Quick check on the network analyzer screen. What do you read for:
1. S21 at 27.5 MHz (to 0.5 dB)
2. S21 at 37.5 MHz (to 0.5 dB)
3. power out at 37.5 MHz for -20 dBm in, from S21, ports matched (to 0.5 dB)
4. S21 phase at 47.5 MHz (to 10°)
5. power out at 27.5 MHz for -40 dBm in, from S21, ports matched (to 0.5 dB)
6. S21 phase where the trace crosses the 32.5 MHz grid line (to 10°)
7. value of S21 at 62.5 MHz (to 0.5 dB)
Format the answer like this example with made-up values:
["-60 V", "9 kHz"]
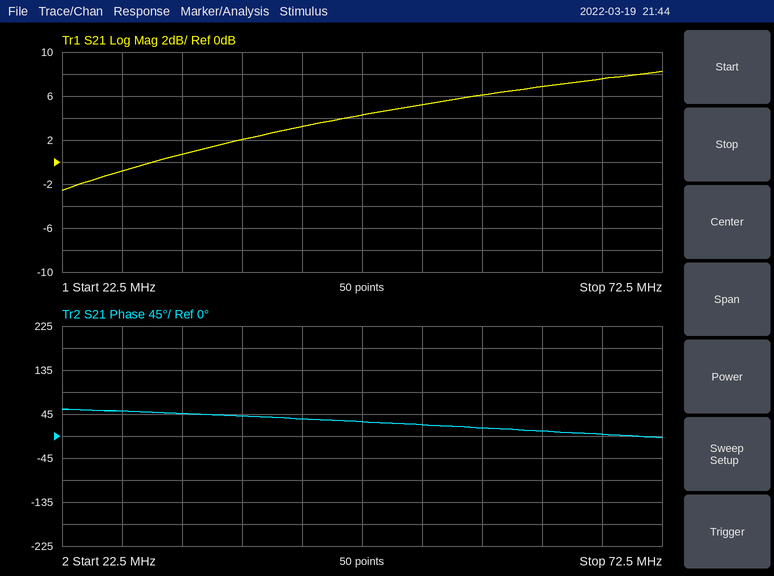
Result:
["-1.0 dB", "2.0 dB", "-18.0 dBm", "30°", "-41.0 dBm", "50°", "7.0 dB"]
